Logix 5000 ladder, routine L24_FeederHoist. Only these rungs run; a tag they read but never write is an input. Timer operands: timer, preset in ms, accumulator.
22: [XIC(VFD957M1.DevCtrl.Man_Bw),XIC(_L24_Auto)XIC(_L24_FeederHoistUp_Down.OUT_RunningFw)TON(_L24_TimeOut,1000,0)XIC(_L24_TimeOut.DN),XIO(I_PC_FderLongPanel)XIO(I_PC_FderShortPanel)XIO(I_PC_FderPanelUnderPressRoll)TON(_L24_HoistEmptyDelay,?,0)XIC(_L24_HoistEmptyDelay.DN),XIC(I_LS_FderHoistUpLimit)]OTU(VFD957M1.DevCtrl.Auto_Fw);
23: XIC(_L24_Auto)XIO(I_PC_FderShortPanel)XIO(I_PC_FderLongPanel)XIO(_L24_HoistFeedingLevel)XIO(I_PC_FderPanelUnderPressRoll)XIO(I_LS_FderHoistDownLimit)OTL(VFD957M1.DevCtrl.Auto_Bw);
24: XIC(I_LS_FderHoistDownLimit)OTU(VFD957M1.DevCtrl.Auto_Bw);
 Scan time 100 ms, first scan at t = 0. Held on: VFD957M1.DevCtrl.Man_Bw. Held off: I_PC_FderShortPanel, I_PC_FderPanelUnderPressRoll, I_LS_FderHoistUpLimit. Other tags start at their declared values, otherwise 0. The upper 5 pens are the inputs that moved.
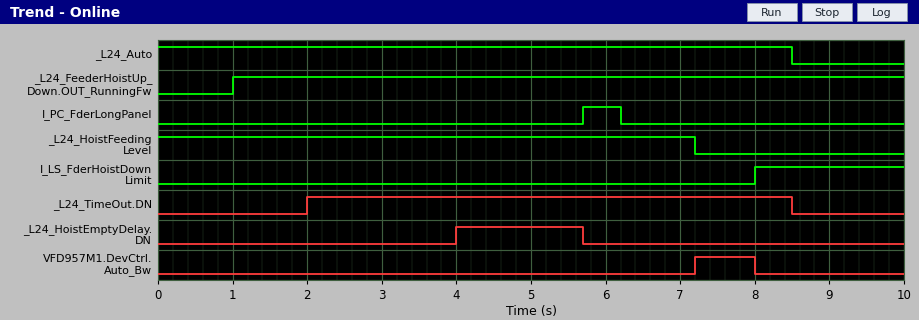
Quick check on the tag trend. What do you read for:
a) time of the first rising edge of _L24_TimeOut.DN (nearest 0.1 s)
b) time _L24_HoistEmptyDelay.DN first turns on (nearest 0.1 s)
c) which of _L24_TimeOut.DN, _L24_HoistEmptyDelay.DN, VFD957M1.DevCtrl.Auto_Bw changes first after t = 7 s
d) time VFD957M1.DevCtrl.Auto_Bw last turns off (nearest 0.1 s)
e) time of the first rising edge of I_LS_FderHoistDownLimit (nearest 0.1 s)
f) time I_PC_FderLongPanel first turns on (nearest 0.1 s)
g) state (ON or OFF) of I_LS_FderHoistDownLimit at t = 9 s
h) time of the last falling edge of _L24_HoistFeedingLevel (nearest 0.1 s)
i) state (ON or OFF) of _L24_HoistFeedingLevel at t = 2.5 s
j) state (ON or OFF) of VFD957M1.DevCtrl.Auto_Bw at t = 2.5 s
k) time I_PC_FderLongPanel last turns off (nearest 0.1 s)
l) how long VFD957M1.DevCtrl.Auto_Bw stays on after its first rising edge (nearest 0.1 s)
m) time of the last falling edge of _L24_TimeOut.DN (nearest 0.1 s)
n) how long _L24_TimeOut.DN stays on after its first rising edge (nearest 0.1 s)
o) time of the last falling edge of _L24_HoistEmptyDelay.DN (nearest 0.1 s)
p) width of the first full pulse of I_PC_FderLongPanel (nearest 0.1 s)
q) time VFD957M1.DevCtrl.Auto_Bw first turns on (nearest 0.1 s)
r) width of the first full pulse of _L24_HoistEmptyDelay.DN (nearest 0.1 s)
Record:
2.0 s
4.0 s
VFD957M1.DevCtrl.Auto_Bw
8.0 s
8.0 s
5.7 s
ON
7.2 s
ON
OFF
6.2 s
0.8 s
8.5 s
6.5 s
5.7 s
0.5 s
7.2 s
1.7 s
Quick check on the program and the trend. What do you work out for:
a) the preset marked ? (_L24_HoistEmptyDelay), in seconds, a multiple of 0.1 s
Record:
4.0 s
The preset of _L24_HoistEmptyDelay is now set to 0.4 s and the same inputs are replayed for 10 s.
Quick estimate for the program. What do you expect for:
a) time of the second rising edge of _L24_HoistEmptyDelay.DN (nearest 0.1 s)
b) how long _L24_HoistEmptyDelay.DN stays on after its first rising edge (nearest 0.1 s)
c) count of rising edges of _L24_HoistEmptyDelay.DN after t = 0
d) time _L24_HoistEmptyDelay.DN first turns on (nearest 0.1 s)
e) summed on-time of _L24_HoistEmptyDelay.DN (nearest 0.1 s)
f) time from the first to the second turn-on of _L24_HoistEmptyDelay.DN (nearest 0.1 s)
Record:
6.6 s
5.3 s
2
0.4 s
8.7 s
6.2 s
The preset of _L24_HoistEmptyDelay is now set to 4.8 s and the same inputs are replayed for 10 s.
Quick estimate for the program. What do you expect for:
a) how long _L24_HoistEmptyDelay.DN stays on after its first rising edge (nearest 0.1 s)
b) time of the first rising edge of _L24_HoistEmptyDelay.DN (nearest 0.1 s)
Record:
0.9 s
4.8 s
